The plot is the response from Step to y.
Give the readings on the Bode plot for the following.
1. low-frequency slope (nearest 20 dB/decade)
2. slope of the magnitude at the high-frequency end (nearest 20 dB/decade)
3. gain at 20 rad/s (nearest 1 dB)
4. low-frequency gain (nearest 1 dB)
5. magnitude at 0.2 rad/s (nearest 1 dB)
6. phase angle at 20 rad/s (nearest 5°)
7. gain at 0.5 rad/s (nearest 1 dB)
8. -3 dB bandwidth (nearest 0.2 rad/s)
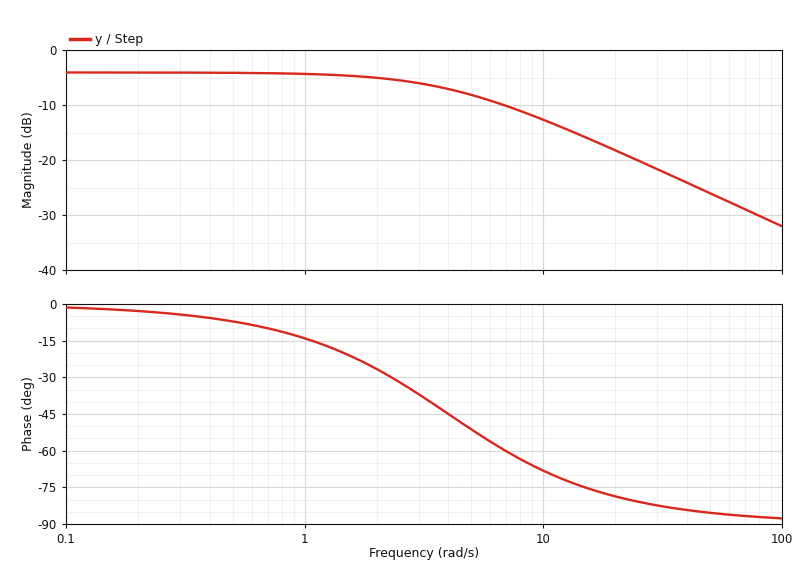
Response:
0 dB/decade
-20 dB/decade
-18 dB
-4 dB
-4 dB
-80°
-4 dB
4.0 rad/s
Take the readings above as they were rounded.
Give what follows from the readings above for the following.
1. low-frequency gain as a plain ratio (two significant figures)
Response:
0.63
